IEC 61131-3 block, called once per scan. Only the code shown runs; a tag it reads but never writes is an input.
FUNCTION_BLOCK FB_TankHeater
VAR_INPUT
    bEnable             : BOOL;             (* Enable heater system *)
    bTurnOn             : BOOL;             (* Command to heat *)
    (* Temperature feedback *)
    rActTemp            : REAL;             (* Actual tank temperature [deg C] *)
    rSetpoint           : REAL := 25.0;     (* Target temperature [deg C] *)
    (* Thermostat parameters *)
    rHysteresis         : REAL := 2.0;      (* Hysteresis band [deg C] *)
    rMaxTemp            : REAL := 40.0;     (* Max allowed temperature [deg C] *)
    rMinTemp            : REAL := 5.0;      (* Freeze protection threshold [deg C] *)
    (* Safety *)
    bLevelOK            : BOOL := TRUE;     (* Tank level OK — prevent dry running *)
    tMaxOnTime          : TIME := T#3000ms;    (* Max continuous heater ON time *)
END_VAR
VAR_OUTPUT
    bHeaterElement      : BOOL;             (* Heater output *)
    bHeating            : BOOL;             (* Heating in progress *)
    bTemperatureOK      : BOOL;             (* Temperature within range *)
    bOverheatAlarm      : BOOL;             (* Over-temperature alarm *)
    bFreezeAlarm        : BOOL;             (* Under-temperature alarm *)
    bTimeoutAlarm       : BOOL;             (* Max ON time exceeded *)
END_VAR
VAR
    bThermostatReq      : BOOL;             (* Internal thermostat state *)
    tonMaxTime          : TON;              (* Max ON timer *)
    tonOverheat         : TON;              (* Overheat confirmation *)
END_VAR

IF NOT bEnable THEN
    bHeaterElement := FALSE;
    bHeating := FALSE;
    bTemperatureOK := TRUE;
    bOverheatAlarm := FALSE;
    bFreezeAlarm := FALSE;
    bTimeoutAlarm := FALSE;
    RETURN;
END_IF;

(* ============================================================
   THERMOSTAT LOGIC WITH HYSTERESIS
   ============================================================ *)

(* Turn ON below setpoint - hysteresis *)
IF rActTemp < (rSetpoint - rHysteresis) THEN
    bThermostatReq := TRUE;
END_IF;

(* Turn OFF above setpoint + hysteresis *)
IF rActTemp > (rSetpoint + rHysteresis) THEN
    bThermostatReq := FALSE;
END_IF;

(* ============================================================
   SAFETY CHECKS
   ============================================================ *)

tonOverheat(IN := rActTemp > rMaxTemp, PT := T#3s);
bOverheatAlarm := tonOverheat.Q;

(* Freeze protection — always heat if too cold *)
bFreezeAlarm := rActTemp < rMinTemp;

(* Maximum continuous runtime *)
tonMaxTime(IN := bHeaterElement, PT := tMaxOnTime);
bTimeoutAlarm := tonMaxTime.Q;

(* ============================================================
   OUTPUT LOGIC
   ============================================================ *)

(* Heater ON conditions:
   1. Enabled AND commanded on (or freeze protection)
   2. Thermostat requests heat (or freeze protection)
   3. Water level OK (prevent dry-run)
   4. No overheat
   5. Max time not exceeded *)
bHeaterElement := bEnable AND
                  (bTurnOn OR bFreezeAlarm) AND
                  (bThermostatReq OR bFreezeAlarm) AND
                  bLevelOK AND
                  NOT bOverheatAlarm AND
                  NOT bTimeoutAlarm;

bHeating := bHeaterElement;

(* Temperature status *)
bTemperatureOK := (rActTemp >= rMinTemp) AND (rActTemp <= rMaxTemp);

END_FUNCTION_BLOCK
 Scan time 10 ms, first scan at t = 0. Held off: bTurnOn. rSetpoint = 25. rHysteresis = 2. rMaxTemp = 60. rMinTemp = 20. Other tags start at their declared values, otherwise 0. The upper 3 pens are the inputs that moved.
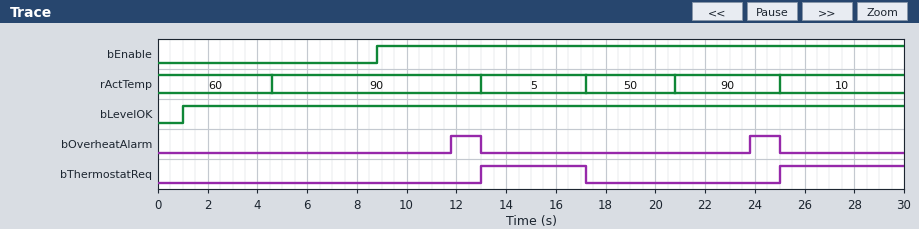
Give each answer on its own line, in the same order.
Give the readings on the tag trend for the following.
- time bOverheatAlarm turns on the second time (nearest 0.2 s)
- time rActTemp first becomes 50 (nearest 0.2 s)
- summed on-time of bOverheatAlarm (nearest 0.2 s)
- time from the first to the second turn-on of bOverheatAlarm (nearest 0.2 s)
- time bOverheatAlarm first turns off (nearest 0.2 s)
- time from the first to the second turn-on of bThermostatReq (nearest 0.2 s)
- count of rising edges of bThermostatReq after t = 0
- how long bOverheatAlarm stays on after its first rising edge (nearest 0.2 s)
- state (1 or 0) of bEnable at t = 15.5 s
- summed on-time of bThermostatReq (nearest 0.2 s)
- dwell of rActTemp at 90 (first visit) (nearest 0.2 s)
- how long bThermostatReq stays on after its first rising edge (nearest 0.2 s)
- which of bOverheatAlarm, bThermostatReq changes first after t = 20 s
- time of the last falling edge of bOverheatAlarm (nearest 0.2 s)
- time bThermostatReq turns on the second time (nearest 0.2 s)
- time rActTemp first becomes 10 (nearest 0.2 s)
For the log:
23.8 s
17.2 s
2.4 s
12.0 s
13.0 s
12.0 s
2
1.2 s
1
9.2 s
8.4 s
4.2 s
bOverheatAlarm
25.0 s
25.0 s
25.0 s
